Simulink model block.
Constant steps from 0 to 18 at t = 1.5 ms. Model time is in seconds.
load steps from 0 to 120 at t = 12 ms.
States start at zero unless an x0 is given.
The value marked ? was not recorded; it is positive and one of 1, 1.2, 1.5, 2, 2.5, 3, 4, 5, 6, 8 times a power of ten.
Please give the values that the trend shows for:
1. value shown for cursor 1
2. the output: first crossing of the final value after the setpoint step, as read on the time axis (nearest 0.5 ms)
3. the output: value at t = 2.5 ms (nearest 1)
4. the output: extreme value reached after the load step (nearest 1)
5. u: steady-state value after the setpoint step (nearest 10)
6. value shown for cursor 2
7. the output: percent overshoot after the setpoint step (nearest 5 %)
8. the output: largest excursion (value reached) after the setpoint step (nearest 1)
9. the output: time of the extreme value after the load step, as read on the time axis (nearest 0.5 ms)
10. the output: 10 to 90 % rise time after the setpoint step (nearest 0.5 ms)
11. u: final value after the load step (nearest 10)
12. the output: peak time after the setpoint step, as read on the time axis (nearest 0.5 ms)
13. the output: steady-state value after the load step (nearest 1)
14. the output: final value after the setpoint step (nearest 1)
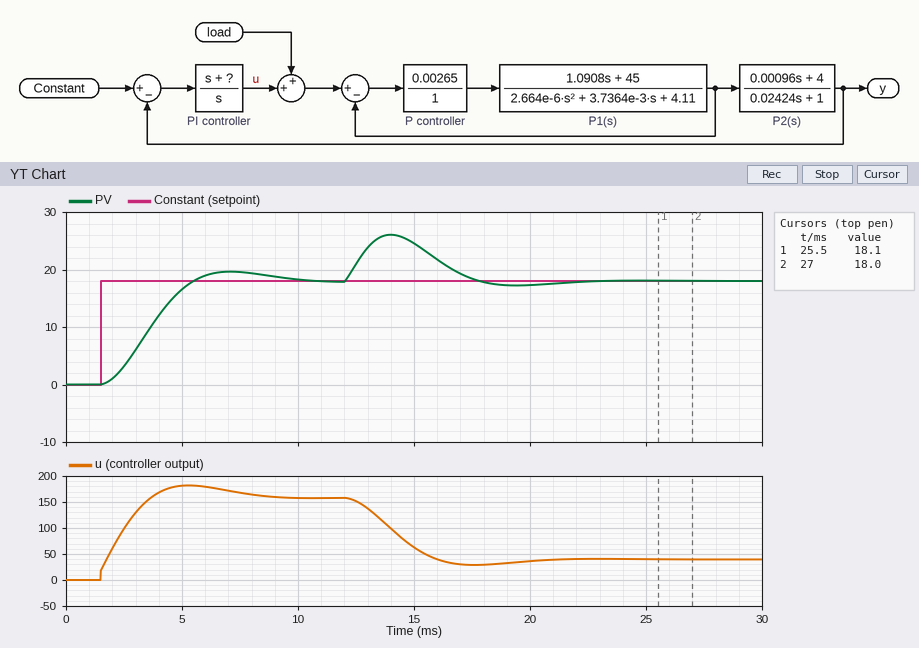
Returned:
18.1
5.5 ms
3
26
160
18.0
10 %
20
14.0 ms
2.5 ms
40
7.0 ms
18
18
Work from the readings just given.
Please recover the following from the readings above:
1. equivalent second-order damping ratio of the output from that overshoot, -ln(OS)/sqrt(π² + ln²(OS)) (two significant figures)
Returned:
0.59
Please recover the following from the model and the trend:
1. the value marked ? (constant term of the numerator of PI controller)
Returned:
5000
